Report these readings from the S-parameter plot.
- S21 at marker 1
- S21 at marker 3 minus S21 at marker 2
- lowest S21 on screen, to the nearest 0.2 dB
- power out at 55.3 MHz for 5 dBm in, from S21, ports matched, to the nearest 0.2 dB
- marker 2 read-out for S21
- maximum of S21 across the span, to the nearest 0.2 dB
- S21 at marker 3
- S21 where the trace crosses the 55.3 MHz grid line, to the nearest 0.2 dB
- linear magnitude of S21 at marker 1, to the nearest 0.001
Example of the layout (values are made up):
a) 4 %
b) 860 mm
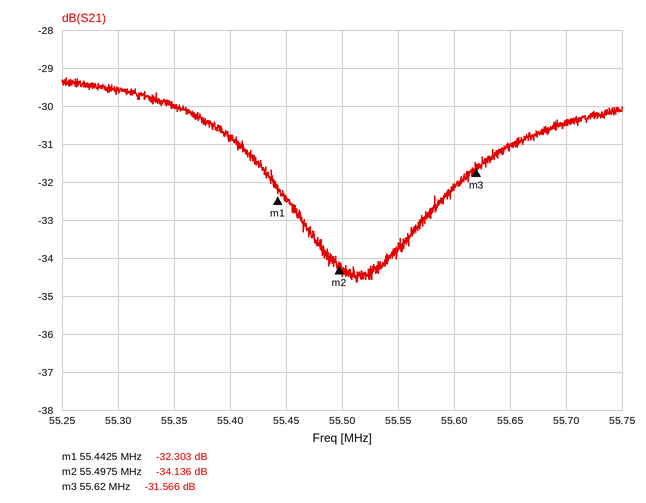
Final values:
a) -32.303 dB
b) 2.570 dB
c) -34.6 dB
d) -24.6 dBm
e) -34.136 dB
f) -29.2 dB
g) -31.566 dB
h) -29.6 dB
i) 0.024
